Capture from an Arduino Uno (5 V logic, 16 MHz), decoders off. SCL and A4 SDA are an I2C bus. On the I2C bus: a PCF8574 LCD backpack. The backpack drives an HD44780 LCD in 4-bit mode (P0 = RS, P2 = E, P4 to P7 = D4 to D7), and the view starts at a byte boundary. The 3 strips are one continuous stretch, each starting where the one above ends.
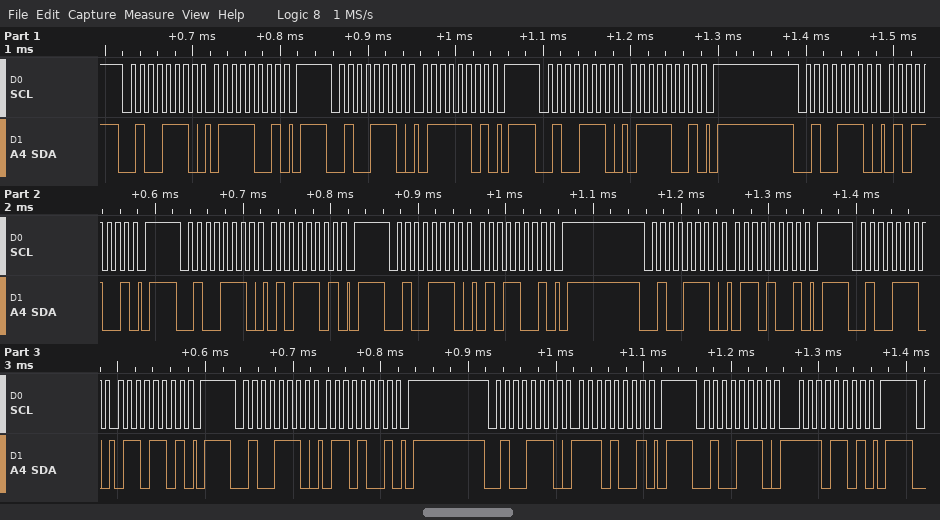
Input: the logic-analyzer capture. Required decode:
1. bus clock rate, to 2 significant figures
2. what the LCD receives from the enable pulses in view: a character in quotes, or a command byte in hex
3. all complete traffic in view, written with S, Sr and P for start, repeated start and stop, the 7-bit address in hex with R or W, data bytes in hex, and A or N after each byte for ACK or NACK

100 kHz
'u'
S 27W A 79 A P S 27W A 7D A P S 27W A 79 A P S 27W A 59 A P S 27W A 5D A P S 27W A 59 A P S 27W A 69 A P S 27W A 6D A P S 27W A 69 A P S 27W A E9 A P S 27W A ED A P
